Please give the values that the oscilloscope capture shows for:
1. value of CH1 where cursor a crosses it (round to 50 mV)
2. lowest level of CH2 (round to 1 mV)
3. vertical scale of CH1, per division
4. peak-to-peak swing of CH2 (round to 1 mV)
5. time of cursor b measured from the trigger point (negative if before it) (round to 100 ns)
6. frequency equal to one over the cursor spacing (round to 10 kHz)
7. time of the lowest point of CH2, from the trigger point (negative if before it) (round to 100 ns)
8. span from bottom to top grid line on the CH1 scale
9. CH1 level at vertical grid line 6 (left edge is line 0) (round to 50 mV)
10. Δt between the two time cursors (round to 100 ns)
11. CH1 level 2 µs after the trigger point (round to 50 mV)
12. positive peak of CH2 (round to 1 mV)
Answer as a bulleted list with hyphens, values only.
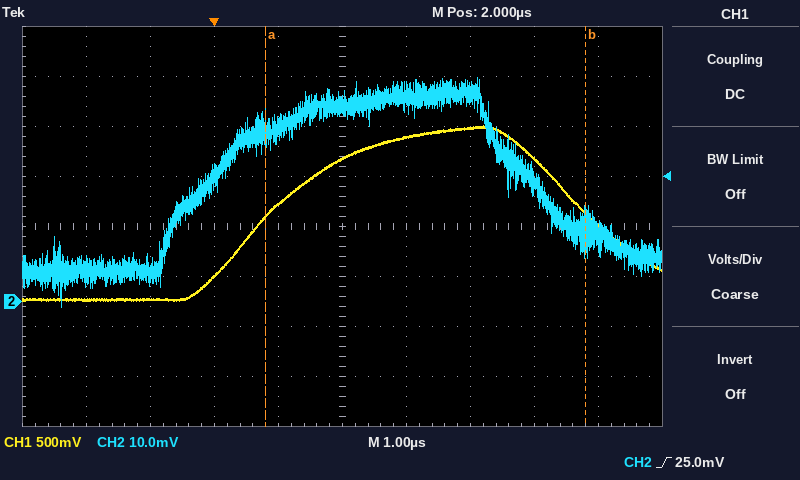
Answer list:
- 850 mV
- -1 mV
- 500 mV
- 46 mV
- +5.8 µs
- 200 kHz
- -2.4 µs
- 4 V
- 1.65 V
- 5.0 µs
- 1.45 V
- 45 mV
